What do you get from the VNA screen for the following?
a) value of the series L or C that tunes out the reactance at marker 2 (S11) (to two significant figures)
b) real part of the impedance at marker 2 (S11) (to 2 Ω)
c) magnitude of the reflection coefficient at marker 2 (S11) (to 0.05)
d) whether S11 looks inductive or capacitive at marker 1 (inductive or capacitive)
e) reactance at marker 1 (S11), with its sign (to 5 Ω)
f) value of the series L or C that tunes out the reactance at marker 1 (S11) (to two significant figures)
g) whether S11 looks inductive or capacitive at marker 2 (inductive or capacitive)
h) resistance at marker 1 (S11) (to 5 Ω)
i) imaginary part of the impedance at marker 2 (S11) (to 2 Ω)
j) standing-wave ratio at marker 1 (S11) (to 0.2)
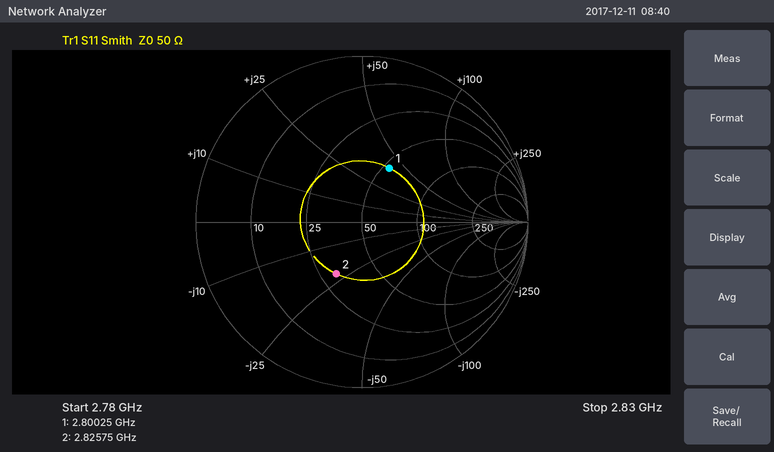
1.2 nH
30 Ω
0.35
inductive
+40 Ω
1.4 pF
capacitive
55 Ω
-22 Ω
2.2
